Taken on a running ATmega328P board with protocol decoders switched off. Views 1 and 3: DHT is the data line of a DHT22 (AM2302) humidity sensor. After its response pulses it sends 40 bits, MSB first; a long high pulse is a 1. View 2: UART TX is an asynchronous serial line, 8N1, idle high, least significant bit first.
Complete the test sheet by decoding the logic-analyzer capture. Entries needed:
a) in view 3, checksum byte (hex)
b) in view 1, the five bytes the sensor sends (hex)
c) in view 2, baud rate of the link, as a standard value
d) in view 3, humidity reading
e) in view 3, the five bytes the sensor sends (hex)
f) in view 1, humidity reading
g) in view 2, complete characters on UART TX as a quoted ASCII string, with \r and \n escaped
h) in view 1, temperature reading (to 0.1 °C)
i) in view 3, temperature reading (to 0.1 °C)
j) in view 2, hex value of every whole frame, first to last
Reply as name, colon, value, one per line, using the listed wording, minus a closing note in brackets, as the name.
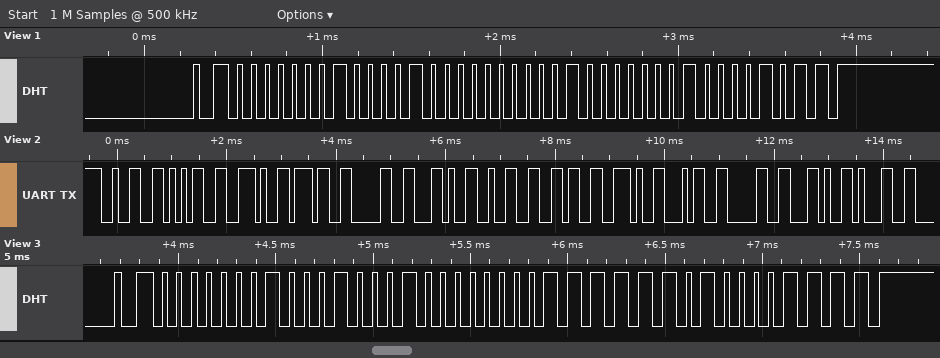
in view 3, checksum byte: 0x0F
in view 1, the five bytes the sensor sends: 01 08 01 01 0B
in view 2, baud rate of the link, as a standard value: 9600 baud
in view 3, humidity reading: 27.3 %
in view 3, the five bytes the sensor sends: 01 11 00 FD 0F
in view 1, humidity reading: 26.4 %
in view 2, complete characters on UART TX as a quoted ASCII string, with \r and \n escaped: "25.70,26.40,1"
in view 1, temperature reading: 25.7 °C
in view 3, temperature reading: 25.3 °C
in view 2, hex value of every whole frame, first to last: 32 35 2E 37 30 2C 32 36 2E 34 30 2C 31
